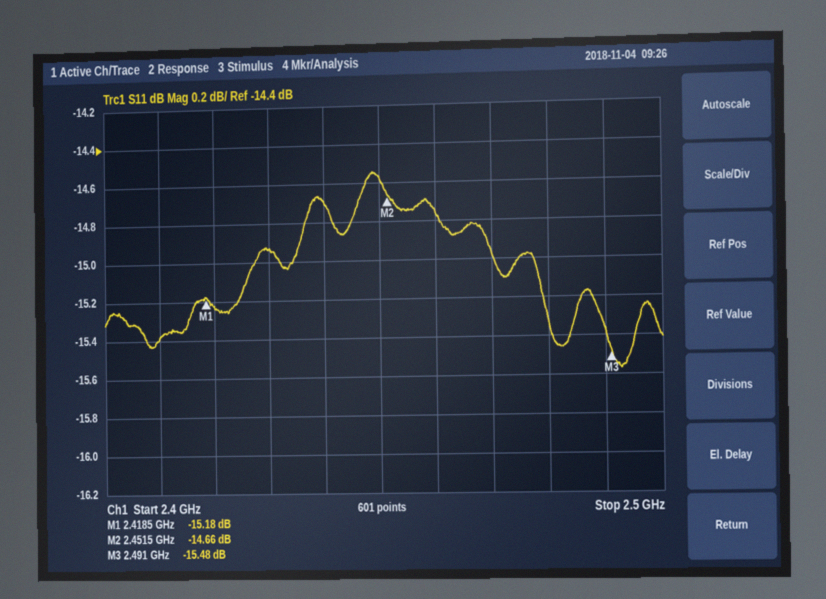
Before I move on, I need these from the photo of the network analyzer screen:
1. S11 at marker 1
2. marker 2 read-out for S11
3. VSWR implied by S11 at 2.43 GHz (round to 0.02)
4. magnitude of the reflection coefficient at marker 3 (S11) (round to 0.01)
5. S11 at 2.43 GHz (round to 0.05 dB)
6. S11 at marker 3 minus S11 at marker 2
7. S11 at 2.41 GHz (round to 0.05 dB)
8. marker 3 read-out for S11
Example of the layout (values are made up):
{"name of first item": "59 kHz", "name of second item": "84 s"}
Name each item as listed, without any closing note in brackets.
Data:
{"S11 at marker 1": "-15.18 dB", "marker 2 read-out for S11": "-14.66 dB", "VSWR implied by S11 at 2.43 GHz": "1.44", "magnitude of the reflection coefficient at marker 3 (S11)": "0.17", "S11 at 2.43 GHz": "-14.95 dB", "S11 at marker 3 minus S11 at marker 2": "-0.82 dB", "S11 at 2.41 GHz": "-15.40 dB", "marker 3 read-out for S11": "-15.48 dB"}
